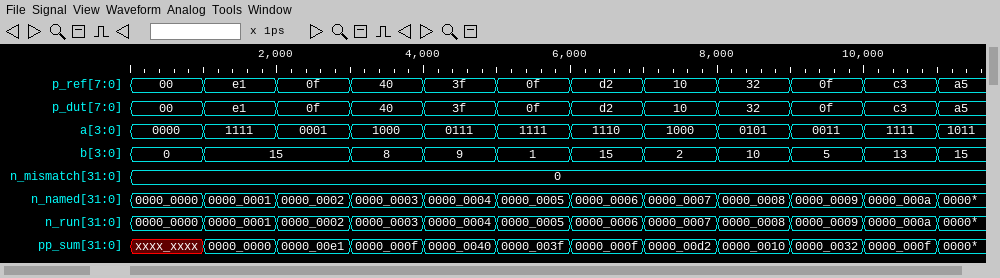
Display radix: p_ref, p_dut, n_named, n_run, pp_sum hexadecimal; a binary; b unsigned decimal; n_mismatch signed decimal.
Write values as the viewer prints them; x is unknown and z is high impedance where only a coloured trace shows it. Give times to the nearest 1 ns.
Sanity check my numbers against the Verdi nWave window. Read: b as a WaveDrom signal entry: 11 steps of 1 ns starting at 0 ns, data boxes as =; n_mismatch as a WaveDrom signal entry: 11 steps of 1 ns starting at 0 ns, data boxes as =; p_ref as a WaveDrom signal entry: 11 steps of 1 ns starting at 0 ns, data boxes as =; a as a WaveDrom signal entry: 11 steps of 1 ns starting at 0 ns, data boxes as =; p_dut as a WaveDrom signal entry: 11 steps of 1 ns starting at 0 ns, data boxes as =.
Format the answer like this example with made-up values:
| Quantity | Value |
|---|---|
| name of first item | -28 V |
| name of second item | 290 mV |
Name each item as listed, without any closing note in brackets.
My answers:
| Quantity | Value |
|---|---|
| b as a WaveDrom signal entry: 11 steps of 1 ns starting at 0 ns, data boxes as = | {name: 'b', wave: '==.========', data: '0 15 8 9 1 15 2 10 5 13'} |
| n_mismatch as a WaveDrom signal entry: 11 steps of 1 ns starting at 0 ns, data boxes as = | {name: 'n_mismatch', wave: '=..........', data: '0'} |
| p_ref as a WaveDrom signal entry: 11 steps of 1 ns starting at 0 ns, data boxes as = | {name: 'p_ref', wave: '===========', data: '00 e1 0f 40 3f 0f d2 10 32 0f c3'} |
| a as a WaveDrom signal entry: 11 steps of 1 ns starting at 0 ns, data boxes as = | {name: 'a', wave: '===========', data: '0000 1111 0001 1000 0111 1111 1110 1000 0101 0011 1111'} |
| p_dut as a WaveDrom signal entry: 11 steps of 1 ns starting at 0 ns, data boxes as = | {name: 'p_dut', wave: '===========', data: '00 e1 0f 40 3f 0f d2 10 32 0f c3'} |
